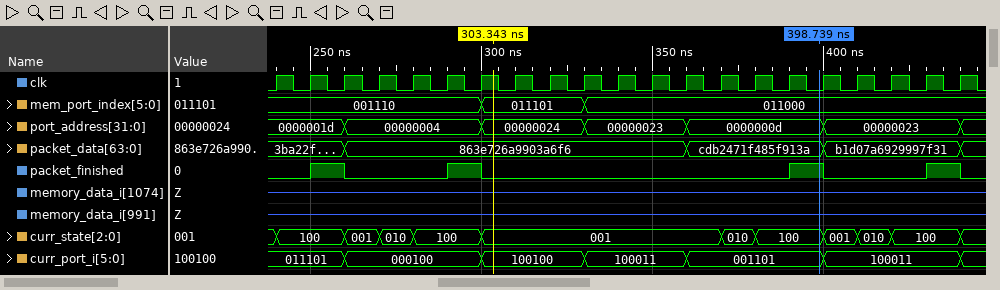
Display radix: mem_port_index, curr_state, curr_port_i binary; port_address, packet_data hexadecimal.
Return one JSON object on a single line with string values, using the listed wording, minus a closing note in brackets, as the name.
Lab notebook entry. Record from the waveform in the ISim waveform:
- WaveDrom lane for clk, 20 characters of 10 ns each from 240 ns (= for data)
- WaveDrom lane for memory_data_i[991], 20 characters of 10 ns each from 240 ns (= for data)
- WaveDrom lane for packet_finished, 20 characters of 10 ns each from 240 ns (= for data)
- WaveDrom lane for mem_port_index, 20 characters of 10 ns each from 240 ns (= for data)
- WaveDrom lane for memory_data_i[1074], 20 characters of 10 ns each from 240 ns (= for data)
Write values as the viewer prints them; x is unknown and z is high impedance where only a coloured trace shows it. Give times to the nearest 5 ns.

{"WaveDrom lane for clk, 20 characters of 10 ns each from 240 ns": "{name: 'clk', wave: 'p...................'}", "WaveDrom lane for memory_data_i[991], 20 characters of 10 ns each from 240 ns": "{name: 'memory_data_i[991]', wave: 'z...................'}", "WaveDrom lane for packet_finished, 20 characters of 10 ns each from 240 ns": "{name: 'packet_finished', wave: '010..10........10..1'}", "WaveDrom lane for mem_port_index, 20 characters of 10 ns each from 240 ns": "{name: 'mem_port_index', wave: '=.....=..=..........', data: '001110 011101 011000'}", "WaveDrom lane for memory_data_i[1074], 20 characters of 10 ns each from 240 ns": "{name: 'memory_data_i[1074]', wave: 'z...................'}"}
